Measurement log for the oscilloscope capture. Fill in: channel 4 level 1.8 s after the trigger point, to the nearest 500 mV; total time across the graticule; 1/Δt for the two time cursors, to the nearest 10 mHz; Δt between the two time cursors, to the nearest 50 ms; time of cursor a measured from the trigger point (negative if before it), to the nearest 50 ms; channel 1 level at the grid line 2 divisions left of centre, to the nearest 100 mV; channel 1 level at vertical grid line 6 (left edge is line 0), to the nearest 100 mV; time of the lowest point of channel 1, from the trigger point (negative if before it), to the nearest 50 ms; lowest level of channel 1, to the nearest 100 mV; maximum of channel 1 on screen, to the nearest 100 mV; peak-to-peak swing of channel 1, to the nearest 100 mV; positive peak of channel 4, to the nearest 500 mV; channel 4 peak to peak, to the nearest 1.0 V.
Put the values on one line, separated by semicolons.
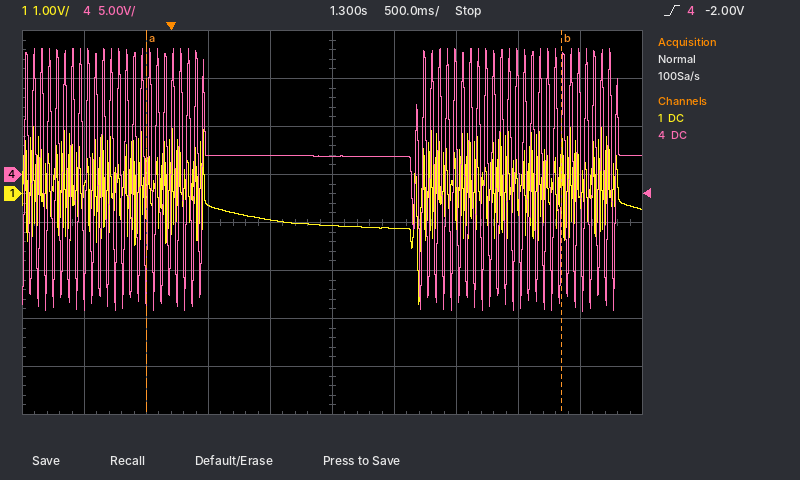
2.0 V; 5 s; 300 mHz; 3.35 s; -200 ms; -200 mV; -700 mV; +2.00 s; -2.3 V; 1.4 V; 3.7 V; 13.0 V; 27.0 V
